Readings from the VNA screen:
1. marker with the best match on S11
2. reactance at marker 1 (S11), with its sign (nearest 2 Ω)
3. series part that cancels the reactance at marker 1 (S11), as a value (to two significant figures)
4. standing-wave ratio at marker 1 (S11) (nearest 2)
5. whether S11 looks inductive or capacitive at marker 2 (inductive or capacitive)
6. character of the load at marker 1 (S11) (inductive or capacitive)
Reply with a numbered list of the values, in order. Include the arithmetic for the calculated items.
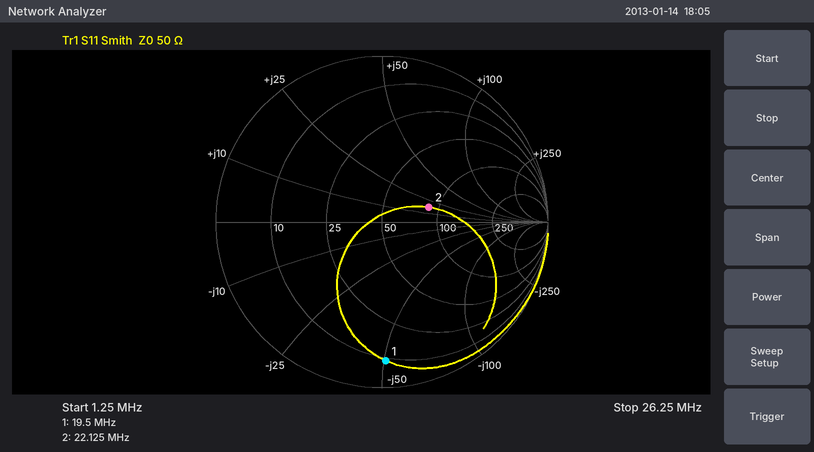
1. marker 2
2. -50 Ω
3. L = 50 Ω/(2π × 19.5 MHz) ≈ 408 nH, so 410 nH to two significant figures
4. 12
5. inductive
6. capacitive
